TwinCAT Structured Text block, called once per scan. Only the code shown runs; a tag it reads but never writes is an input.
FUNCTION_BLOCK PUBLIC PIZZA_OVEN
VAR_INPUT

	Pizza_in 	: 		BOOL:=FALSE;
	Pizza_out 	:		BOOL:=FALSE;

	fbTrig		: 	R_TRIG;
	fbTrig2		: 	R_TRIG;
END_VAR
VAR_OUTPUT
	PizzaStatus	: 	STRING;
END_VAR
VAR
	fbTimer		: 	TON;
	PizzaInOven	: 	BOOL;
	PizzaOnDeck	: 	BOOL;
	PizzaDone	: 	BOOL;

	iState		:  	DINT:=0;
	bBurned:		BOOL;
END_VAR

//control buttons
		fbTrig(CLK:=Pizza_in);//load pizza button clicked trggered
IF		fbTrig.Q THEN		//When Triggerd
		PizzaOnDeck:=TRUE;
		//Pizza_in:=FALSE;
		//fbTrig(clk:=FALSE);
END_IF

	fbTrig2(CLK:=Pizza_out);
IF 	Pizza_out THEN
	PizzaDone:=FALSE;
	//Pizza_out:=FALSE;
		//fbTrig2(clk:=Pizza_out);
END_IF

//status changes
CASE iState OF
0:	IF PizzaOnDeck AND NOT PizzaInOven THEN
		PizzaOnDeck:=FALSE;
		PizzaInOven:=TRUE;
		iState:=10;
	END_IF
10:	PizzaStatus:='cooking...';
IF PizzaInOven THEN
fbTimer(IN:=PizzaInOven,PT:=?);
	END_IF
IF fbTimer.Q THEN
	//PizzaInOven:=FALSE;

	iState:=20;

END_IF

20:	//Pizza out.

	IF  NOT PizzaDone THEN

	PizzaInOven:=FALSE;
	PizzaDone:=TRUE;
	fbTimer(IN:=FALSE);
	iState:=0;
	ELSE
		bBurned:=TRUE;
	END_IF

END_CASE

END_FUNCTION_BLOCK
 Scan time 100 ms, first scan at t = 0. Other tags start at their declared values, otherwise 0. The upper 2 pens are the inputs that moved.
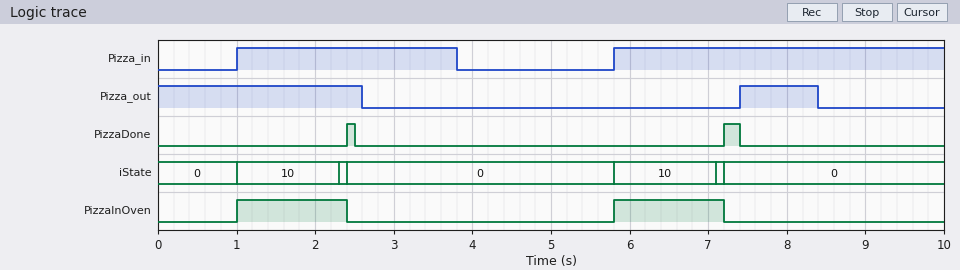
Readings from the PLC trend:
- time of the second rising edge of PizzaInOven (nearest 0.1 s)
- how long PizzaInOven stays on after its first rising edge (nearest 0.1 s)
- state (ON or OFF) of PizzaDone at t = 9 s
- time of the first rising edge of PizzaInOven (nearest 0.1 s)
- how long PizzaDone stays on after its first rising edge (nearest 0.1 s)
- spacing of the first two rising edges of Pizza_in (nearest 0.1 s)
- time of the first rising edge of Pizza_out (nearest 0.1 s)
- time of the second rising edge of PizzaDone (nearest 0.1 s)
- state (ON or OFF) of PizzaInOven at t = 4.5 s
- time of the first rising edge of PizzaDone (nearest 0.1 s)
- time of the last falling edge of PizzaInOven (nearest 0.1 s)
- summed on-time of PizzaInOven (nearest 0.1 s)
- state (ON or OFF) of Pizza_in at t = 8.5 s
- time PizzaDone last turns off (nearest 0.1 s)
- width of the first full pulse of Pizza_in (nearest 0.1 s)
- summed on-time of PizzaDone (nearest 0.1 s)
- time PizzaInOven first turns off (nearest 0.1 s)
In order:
5.8 s
1.4 s
OFF
1.0 s
0.1 s
4.8 s
7.4 s
7.2 s
OFF
2.4 s
7.2 s
2.8 s
ON
7.4 s
2.8 s
0.3 s
2.4 s
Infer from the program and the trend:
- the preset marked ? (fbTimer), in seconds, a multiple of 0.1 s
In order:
1.2 s
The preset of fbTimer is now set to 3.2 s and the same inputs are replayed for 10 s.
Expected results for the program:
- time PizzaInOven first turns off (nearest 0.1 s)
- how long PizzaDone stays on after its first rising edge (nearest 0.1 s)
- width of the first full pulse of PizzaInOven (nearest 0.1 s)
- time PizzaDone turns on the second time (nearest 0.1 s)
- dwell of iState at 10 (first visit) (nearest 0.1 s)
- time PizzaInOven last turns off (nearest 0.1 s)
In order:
4.4 s
3.0 s
3.4 s
9.2 s
3.3 s
9.2 s
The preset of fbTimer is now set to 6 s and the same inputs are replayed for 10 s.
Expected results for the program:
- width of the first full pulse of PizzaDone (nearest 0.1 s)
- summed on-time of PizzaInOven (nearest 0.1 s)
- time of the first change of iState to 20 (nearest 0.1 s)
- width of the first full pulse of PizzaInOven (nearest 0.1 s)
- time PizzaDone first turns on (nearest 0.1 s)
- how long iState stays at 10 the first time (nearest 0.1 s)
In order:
0.2 s
8.9 s
7.1 s
6.2 s
7.2 s
6.1 s
